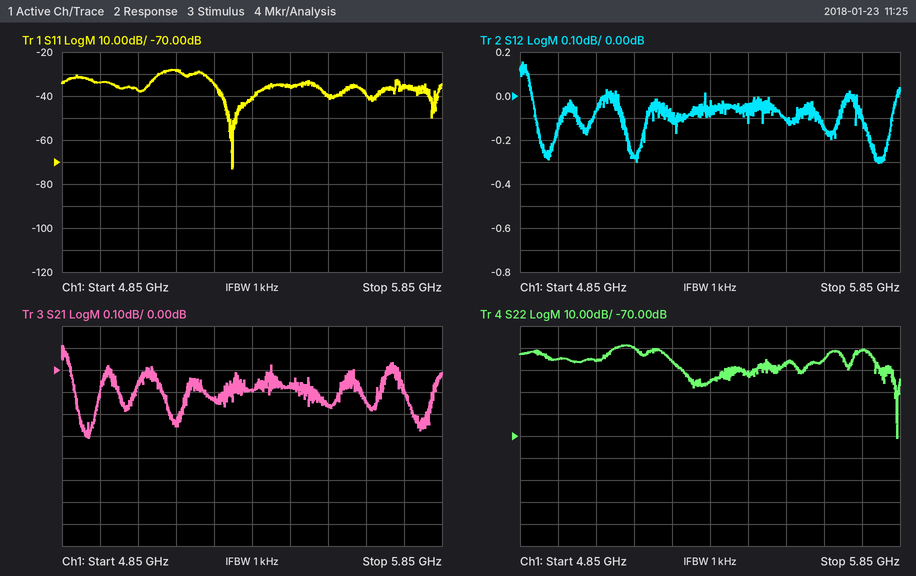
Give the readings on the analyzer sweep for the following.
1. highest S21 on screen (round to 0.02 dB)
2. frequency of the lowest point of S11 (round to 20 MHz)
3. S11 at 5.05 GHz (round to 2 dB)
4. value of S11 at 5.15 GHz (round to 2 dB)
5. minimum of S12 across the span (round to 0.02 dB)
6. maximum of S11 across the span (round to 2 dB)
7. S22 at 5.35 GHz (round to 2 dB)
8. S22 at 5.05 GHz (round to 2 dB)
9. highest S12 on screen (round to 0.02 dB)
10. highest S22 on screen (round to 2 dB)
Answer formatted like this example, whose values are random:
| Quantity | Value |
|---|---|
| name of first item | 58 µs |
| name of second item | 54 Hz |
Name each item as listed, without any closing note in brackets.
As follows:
| Quantity | Value |
|---|---|
| highest S21 on screen | 0.12 dB |
| frequency of the lowest point of S11 | 5.30 GHz |
| S11 at 5.05 GHz | -38 dB |
| value of S11 at 5.15 GHz | -28 dB |
| minimum of S12 across the span | -0.30 dB |
| maximum of S11 across the span | -28 dB |
| S22 at 5.35 GHz | -46 dB |
| S22 at 5.05 GHz | -36 dB |
| highest S12 on screen | 0.16 dB |
| highest S22 on screen | -28 dB |
